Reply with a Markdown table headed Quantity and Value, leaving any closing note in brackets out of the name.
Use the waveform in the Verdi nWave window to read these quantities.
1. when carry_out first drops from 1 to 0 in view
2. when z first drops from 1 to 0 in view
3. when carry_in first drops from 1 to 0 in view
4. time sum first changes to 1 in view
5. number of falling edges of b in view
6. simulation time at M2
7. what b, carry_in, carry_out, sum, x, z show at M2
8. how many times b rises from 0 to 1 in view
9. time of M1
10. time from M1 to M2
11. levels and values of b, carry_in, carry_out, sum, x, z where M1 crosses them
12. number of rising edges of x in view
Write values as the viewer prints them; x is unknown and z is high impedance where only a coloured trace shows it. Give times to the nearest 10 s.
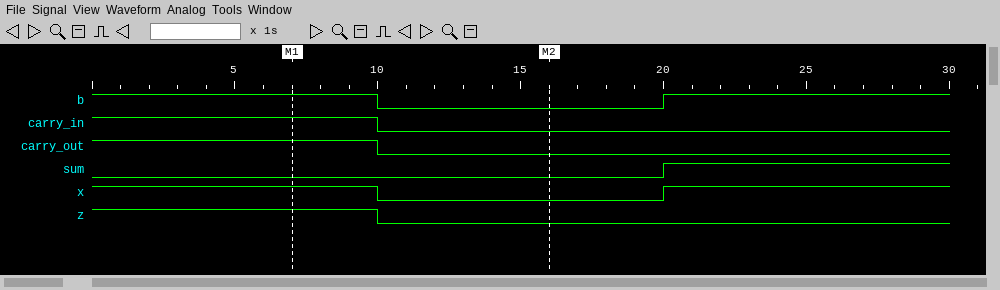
| Quantity | Value |
|---|---|
| when carry_out first drops from 1 to 0 in view | 10 s |
| when z first drops from 1 to 0 in view | 10 s |
| when carry_in first drops from 1 to 0 in view | 10 s |
| time sum first changes to 1 in view | 20 s |
| number of falling edges of b in view | 1 |
| simulation time at M2 | 20 s |
| what b, carry_in, carry_out, sum, x, z show at M2 | b=0, carry_in=0, carry_out=0, sum=0, x=0, z=0 |
| how many times b rises from 0 to 1 in view | 1 |
| time of M1 | 10 s |
| time from M1 to M2 | 10 s |
| levels and values of b, carry_in, carry_out, sum, x, z where M1 crosses them | b=1, carry_in=1, carry_out=1, sum=0, x=1, z=1 |
| number of rising edges of x in view | 1 |
